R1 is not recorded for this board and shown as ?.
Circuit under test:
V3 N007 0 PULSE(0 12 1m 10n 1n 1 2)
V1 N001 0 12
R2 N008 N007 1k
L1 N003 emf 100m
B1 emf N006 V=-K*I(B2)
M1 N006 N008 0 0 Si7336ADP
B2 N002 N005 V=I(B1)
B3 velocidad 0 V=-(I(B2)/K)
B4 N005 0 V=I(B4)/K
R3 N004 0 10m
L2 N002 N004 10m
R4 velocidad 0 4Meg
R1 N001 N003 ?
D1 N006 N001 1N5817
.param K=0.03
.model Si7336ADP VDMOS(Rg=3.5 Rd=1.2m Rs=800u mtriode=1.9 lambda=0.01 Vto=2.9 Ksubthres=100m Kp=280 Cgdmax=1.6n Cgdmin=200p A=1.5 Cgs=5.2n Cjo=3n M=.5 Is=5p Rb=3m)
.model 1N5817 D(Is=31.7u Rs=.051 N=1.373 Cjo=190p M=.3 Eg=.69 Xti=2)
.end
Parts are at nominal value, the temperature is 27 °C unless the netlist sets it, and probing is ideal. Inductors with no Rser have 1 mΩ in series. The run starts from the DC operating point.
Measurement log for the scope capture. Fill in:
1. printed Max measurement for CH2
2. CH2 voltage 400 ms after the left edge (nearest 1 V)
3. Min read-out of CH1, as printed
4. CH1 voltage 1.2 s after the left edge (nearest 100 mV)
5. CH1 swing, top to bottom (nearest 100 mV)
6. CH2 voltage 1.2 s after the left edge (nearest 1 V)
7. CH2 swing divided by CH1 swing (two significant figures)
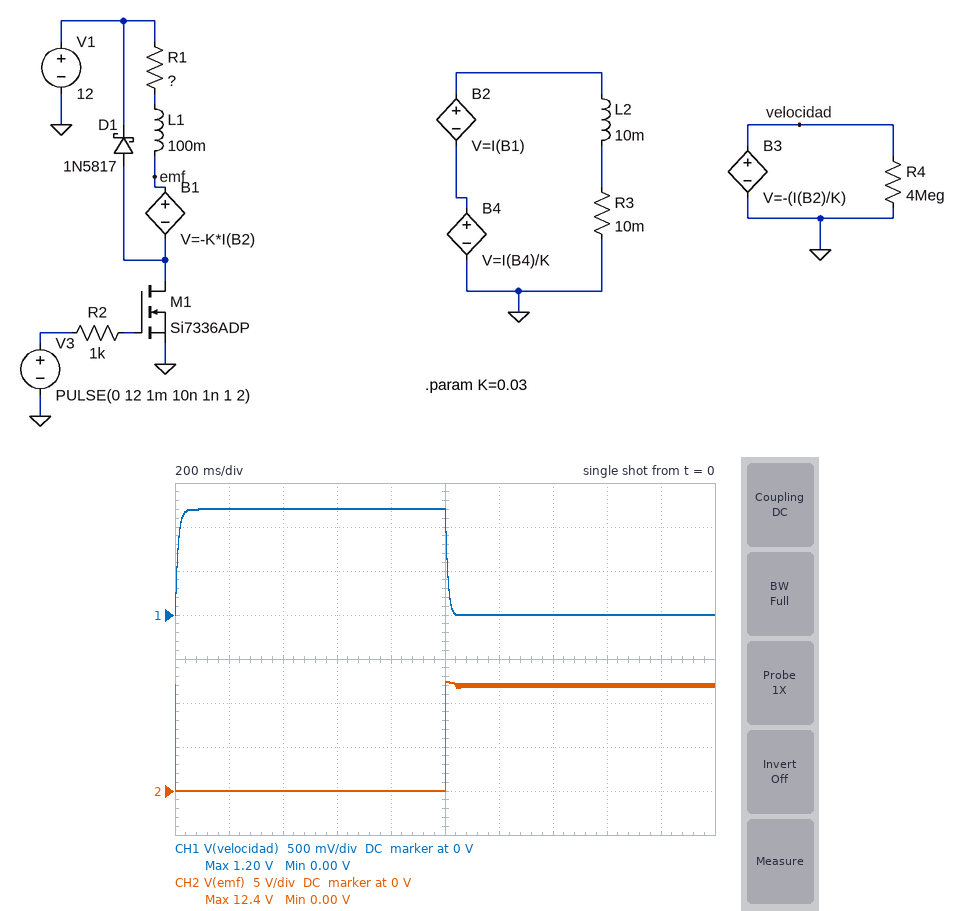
12.4 V
0 V
0.00 V
0 V
1.2 V
12 V
10
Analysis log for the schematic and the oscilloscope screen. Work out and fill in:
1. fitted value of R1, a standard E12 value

10 Ω
